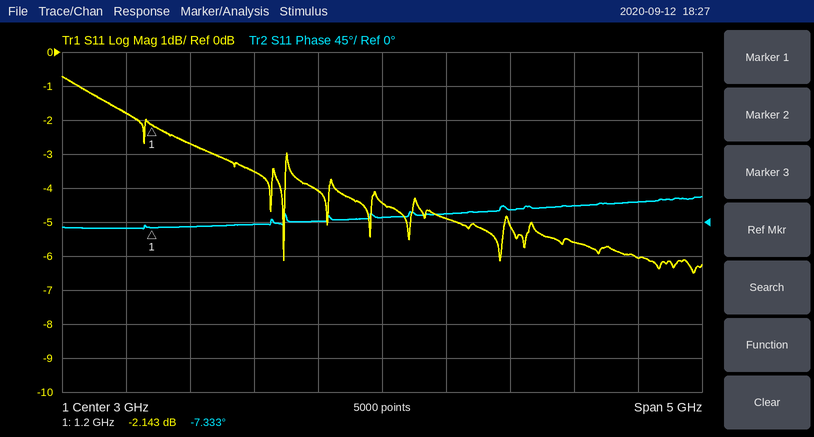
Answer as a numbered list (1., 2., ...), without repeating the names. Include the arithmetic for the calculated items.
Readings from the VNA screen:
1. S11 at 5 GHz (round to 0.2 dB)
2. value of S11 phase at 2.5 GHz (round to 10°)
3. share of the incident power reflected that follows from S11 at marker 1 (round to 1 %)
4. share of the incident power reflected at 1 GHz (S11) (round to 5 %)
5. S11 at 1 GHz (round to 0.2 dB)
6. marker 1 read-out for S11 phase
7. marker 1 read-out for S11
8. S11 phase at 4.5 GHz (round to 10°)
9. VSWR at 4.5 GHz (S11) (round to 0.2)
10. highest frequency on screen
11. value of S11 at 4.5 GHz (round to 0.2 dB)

1. -6.0 dB
2. 0°
3. 10^(-2.143/10) ≈ 61 %
4. 10^(-1.8/10) ≈ 66.1 %, so 65 % to the nearest 5 %
5. -1.8 dB
6. -7.333°
7. -2.143 dB
8. 20°
9. |Γ| = 10^(-5.6/20) = 0.5248; VSWR = (1 + 0.5248)/(1 − 0.5248) ≈ 3.2
10. 5.5 GHz
11. -5.6 dB
